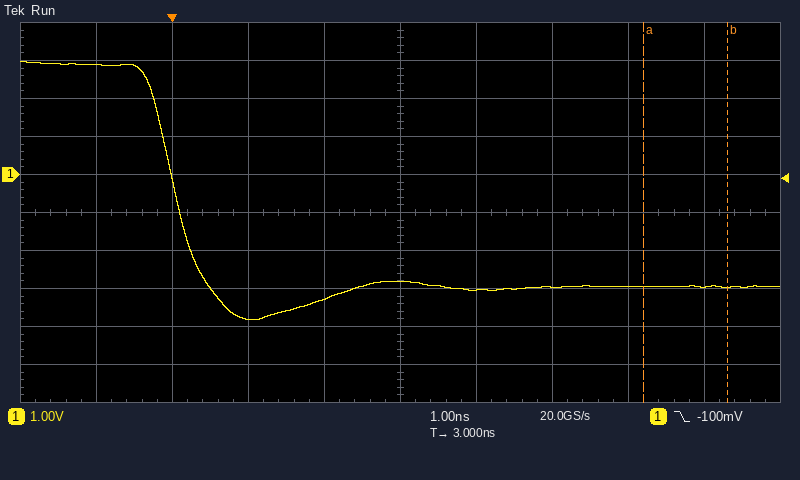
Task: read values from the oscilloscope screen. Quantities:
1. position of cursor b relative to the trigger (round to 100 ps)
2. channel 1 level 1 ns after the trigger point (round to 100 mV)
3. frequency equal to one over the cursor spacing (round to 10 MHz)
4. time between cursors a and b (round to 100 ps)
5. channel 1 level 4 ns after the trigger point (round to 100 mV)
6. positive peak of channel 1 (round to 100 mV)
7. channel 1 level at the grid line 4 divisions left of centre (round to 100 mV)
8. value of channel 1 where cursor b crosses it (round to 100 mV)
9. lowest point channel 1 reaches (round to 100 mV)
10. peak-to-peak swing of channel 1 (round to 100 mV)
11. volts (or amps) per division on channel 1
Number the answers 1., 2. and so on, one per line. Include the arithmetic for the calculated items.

1. +7.3 ns
2. -3.8 V
3. 1 / 1.1 ns ≈ 910 MHz
4. 1.1 ns
5. -3.0 V
6. 3.0 V
7. 2.9 V
8. -3.0 V
9. -3.8 V
10. 3.0 V − (-3.8 V) = 6.8 V
11. 1 V
